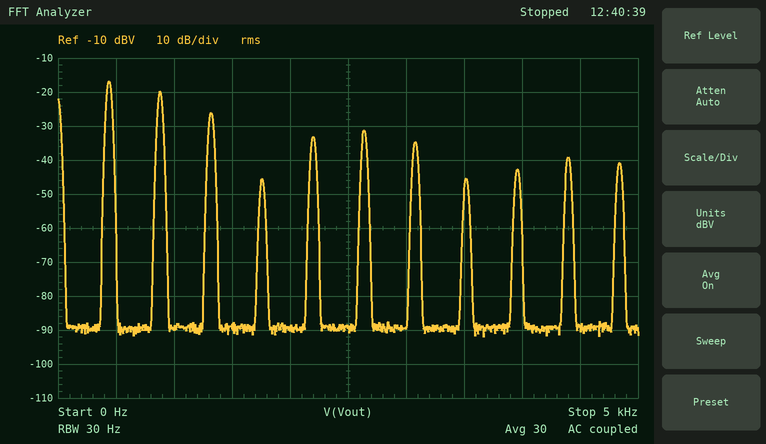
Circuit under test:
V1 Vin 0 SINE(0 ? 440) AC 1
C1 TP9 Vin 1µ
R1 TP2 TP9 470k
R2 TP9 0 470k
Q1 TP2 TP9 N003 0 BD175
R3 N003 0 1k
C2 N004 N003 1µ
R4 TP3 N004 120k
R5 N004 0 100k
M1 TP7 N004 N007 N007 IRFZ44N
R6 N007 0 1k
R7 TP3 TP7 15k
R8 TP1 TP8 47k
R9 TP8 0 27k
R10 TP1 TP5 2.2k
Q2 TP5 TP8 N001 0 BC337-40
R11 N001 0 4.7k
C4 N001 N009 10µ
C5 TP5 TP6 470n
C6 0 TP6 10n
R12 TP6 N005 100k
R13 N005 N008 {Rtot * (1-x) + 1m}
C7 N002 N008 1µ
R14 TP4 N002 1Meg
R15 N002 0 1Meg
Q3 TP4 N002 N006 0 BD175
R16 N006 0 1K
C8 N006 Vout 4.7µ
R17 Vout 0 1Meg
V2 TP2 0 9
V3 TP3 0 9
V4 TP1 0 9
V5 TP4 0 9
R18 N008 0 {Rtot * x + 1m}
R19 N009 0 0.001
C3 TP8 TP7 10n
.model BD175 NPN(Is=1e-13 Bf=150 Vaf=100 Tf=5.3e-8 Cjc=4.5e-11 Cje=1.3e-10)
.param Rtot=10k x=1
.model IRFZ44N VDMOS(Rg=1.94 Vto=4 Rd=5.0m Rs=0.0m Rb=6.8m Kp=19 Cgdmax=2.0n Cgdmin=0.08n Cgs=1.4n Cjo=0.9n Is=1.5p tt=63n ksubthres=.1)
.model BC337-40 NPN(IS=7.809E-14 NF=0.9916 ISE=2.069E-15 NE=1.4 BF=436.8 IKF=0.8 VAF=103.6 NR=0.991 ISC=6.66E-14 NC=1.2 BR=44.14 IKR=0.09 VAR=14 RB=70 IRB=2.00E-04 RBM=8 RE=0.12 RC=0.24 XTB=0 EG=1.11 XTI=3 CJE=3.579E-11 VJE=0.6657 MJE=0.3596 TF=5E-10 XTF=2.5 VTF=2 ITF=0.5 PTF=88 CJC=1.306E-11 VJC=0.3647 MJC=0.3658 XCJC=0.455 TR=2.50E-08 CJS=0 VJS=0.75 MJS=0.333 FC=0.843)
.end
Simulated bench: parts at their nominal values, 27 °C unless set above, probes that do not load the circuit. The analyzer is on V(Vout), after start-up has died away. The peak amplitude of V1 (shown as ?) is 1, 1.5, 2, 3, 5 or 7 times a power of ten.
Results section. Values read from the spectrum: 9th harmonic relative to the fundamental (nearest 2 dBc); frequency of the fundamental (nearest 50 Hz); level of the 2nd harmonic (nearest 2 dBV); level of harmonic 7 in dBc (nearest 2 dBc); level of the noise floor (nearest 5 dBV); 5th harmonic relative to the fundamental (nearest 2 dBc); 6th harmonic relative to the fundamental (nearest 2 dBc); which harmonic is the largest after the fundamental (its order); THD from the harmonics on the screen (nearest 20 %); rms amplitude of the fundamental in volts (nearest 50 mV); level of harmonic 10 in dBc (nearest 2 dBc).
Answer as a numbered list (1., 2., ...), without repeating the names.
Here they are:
1. -26 dBc
2. 450 Hz
3. -20 dBV
4. -18 dBc
5. -90 dBV
6. -16 dBc
7. -14 dBc
8. 2
9. 80 %
10. 150 mV
11. -22 dBc
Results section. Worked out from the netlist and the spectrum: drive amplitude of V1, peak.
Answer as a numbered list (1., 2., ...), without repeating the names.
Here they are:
1. 150 mV
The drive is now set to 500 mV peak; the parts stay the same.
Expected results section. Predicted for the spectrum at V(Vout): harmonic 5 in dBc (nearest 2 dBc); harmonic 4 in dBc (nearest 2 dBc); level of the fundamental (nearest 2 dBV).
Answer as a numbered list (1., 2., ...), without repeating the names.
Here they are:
1. -12 dBc
2. -20 dBc
3. -16 dBV
